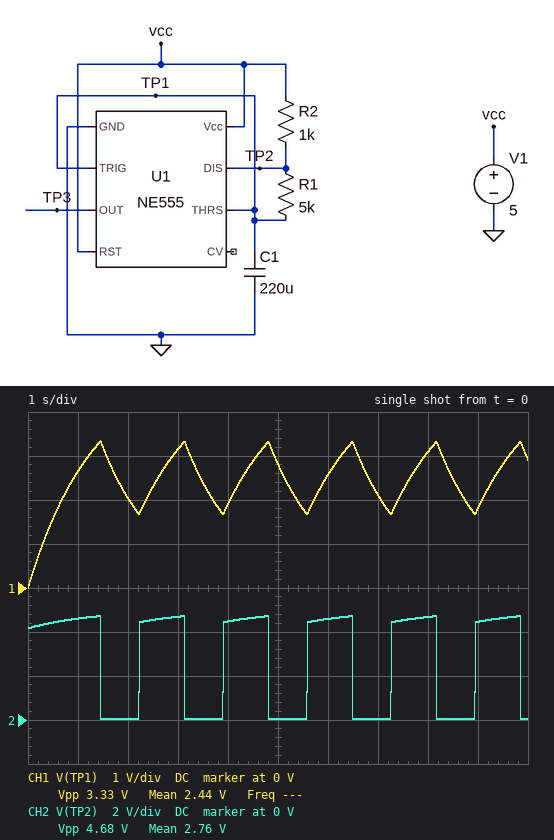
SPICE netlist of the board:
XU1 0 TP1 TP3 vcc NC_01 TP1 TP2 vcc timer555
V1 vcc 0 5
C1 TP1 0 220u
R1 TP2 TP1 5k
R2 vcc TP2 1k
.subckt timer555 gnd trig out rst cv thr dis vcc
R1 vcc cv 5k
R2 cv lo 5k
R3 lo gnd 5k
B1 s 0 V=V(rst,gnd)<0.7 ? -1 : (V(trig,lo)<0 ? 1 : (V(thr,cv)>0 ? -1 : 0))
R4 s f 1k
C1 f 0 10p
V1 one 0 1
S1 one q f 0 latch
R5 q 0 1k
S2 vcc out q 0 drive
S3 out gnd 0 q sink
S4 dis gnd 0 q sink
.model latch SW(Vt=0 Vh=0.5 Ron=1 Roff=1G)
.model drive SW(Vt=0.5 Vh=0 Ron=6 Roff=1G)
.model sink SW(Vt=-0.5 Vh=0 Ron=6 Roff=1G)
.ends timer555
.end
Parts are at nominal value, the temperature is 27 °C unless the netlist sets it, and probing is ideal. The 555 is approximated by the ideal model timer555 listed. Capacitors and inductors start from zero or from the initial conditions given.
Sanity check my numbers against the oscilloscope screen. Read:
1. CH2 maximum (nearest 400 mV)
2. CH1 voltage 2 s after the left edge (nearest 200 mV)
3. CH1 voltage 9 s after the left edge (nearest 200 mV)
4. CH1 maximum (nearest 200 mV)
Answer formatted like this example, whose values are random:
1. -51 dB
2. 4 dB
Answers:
1. 4.8 V
2. 2.0 V
3. 1.8 V
4. 3.4 V
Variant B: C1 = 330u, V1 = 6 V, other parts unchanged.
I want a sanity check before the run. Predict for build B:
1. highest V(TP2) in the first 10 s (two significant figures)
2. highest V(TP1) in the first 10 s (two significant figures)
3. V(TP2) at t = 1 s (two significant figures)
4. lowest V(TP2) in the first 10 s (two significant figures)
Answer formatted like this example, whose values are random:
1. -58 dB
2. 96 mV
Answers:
1. 5.7 V
2. 4.0 V
3. 5.4 V
4. 38 mV
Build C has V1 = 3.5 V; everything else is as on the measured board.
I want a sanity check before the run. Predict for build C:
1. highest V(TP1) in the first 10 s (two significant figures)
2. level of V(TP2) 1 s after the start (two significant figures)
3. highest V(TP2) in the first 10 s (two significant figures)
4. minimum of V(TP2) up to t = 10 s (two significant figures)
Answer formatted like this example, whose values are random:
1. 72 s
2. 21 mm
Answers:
1. 2.3 V
2. 3.2 V
3. 3.3 V
4. 22 mV
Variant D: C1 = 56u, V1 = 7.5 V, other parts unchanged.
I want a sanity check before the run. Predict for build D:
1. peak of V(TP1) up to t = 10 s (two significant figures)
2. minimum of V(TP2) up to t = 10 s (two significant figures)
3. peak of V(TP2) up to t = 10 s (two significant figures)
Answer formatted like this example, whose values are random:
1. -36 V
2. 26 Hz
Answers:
1. 5.0 V
2. 48 mV
3. 7.1 V
